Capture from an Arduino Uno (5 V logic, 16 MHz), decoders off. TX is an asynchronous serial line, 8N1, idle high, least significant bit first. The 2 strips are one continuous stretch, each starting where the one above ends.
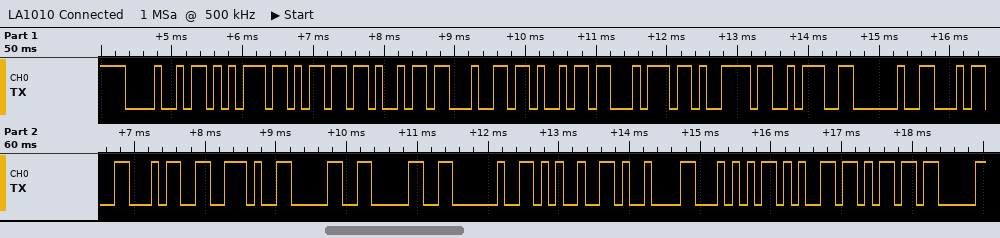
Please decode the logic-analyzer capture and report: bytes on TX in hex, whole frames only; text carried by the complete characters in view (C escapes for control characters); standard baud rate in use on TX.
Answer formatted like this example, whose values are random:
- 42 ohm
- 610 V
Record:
- 48 75 6D 69 64 69 74 79 3A 20 34 34 2E 30 30 20 25 09 54 65 6D
- "Humidity: 44.00 %\tTem"
- 9600 baud
